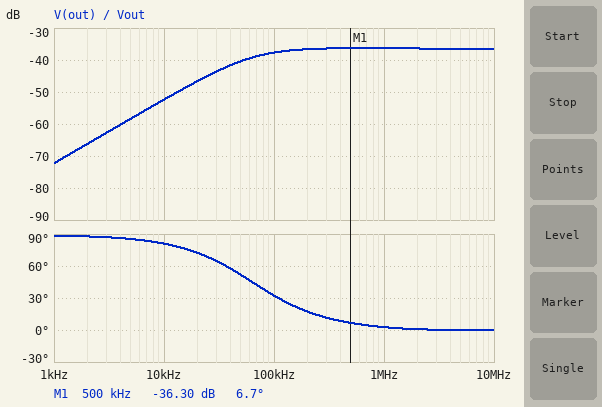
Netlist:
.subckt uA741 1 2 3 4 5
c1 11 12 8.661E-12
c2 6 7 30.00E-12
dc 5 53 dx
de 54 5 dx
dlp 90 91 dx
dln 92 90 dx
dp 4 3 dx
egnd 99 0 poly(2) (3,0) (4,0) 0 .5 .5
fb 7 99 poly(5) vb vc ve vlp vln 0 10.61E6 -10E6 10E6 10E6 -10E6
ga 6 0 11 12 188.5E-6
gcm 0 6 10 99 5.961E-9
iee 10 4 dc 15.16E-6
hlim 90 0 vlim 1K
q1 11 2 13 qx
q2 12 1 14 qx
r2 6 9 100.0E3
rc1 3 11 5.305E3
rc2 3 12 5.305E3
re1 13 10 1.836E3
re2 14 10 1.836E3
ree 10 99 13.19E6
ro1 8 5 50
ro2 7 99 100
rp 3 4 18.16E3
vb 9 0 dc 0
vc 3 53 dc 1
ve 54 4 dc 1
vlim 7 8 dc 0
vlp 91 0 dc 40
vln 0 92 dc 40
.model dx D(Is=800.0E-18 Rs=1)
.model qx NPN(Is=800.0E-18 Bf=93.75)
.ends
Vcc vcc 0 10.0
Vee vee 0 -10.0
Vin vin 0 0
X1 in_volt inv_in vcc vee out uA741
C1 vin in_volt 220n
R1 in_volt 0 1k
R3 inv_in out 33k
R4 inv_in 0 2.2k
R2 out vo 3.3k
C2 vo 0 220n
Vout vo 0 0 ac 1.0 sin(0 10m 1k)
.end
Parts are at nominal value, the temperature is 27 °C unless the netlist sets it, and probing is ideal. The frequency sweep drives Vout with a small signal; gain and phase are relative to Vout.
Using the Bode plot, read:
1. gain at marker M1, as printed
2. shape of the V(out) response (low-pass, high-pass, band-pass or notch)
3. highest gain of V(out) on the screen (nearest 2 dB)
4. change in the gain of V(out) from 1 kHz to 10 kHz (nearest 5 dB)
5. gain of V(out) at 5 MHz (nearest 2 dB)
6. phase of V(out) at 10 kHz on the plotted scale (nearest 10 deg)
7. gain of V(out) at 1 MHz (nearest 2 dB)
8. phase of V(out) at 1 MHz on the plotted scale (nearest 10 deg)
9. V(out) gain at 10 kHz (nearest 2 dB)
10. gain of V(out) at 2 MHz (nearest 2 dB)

-36.30 dB
high-pass
-36 dB
20 dB
-36 dB
80 deg
-36 dB
0 deg
-52 dB
-36 dB
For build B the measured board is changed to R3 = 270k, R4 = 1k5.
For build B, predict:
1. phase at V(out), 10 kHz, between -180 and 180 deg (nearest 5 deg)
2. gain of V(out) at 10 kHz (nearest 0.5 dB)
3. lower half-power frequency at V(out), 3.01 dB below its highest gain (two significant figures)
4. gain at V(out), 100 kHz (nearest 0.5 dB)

30 deg
-37.5 dB
5.4 kHz
-36.5 dB
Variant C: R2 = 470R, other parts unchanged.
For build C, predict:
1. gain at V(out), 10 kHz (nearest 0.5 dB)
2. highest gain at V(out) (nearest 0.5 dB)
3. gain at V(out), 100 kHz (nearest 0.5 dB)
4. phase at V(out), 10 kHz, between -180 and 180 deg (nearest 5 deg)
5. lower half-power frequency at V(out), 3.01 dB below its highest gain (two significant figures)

-35.5 dB
-20.0 dB
-21.5 dB
80 deg
57 kHz
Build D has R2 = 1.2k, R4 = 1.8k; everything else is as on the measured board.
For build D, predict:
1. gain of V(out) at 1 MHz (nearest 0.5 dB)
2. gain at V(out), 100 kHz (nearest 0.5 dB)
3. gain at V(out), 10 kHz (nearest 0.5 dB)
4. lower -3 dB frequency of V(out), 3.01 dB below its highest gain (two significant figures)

-28.0 dB
-28.5 dB
-42.0 dB
50 kHz
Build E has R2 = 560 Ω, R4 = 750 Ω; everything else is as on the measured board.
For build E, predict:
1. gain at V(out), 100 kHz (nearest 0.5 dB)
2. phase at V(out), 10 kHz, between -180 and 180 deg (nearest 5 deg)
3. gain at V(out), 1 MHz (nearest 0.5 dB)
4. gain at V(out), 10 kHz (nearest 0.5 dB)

-22.0 dB
65 deg
-21.5 dB
-29.0 dB
